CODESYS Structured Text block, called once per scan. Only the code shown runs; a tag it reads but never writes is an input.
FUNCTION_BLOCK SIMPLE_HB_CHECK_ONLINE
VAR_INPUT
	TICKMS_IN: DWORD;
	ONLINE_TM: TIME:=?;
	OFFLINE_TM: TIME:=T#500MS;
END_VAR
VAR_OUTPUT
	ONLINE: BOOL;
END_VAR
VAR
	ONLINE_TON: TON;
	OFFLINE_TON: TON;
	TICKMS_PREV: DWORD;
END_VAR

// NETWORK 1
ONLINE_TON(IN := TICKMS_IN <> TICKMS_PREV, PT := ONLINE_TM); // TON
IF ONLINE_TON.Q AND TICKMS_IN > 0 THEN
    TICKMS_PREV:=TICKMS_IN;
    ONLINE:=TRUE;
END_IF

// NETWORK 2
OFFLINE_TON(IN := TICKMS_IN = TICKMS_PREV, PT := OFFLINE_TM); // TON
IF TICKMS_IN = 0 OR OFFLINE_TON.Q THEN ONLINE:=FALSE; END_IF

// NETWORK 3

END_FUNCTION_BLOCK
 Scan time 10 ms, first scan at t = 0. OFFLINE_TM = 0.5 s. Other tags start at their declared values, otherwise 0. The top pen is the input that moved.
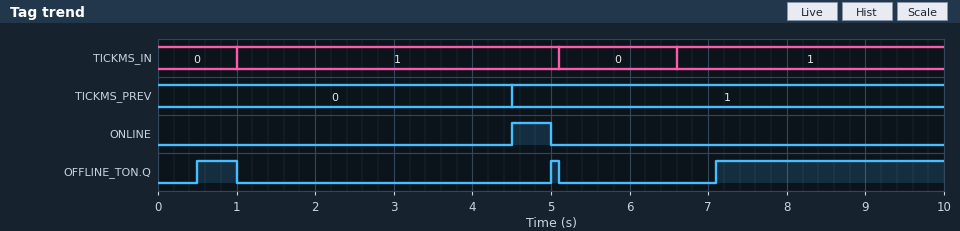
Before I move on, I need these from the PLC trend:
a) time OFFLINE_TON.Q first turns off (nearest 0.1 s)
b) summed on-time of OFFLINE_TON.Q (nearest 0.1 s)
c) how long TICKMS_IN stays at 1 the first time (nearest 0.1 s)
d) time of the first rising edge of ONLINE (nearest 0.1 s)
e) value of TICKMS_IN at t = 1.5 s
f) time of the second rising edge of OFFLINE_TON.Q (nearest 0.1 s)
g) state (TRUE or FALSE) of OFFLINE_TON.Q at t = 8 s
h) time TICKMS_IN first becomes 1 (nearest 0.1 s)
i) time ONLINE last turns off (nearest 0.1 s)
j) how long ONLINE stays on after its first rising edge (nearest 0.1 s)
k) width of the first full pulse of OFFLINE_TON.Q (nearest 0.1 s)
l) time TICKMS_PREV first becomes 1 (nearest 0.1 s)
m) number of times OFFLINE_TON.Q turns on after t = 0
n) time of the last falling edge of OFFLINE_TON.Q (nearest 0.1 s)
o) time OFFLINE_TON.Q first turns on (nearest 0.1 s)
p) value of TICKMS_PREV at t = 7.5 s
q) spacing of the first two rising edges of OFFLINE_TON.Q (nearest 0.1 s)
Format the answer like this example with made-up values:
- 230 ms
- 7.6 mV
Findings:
- 1.0 s
- 3.5 s
- 4.1 s
- 4.5 s
- 1
- 5.0 s
- TRUE
- 1.0 s
- 5.0 s
- 0.5 s
- 0.5 s
- 4.5 s
- 3
- 5.1 s
- 0.5 s
- 1
- 4.5 s
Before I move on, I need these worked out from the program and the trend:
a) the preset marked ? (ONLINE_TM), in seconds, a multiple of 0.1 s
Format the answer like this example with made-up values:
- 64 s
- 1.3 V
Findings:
- 3.5 s
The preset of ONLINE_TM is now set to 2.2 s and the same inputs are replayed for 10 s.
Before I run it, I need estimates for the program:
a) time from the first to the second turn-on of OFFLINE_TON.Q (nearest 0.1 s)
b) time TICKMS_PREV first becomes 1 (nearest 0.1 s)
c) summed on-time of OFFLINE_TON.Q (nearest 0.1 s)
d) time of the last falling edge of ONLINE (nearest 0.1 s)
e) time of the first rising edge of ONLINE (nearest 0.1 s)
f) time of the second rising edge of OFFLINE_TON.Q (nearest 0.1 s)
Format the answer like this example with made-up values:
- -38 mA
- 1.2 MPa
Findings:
- 3.2 s
- 3.2 s
- 4.8 s
- 3.7 s
- 3.2 s
- 3.7 s
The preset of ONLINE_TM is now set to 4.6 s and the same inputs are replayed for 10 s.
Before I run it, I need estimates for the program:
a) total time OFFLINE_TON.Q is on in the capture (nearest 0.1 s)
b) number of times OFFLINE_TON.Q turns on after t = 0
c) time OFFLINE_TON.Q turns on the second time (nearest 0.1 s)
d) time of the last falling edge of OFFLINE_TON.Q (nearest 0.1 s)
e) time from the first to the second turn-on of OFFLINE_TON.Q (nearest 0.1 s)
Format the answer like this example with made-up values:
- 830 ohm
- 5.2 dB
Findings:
- 1.5 s
- 2
- 5.6 s
- 6.6 s
- 5.1 s
